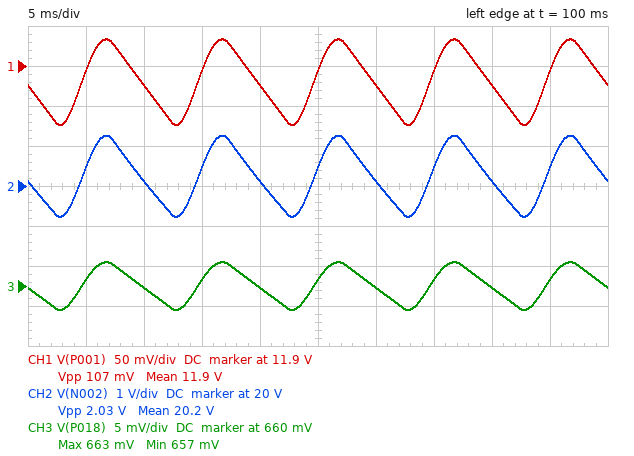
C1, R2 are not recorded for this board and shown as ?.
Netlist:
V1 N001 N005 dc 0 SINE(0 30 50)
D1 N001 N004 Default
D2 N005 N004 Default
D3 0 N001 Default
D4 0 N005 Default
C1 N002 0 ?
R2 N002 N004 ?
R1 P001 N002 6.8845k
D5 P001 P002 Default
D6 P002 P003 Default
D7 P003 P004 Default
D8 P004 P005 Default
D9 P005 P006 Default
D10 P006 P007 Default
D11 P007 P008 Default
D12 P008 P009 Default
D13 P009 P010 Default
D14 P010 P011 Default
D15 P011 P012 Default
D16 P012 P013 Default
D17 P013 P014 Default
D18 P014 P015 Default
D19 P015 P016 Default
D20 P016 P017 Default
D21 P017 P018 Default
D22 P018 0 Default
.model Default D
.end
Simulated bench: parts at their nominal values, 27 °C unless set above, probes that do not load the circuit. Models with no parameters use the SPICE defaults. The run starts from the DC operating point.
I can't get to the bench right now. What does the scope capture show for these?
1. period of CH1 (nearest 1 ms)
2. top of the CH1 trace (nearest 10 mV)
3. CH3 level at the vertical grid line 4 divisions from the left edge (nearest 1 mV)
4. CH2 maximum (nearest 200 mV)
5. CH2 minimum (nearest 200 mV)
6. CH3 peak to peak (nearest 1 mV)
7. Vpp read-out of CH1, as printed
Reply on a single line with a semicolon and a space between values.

10 ms; 11.93 V; 660 mV; 21.2 V; 19.2 V; 6 mV; 107 mV
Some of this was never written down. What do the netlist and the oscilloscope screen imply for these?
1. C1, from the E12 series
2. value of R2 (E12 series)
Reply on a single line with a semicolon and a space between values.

3.3 µF; 2.2 kΩ
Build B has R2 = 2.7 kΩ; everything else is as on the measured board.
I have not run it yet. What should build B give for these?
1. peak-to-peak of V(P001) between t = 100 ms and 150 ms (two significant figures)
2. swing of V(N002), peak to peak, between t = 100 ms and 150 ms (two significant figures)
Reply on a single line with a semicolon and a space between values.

100 mV; 1.8 V
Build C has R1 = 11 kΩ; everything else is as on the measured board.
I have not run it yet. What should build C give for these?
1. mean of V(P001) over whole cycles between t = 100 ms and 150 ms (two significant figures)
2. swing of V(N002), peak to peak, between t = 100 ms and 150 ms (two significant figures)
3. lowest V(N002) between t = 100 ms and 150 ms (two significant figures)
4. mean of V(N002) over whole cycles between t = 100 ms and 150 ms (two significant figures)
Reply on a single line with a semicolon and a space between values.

12 V; 1.6 V; 21 V; 22 V
